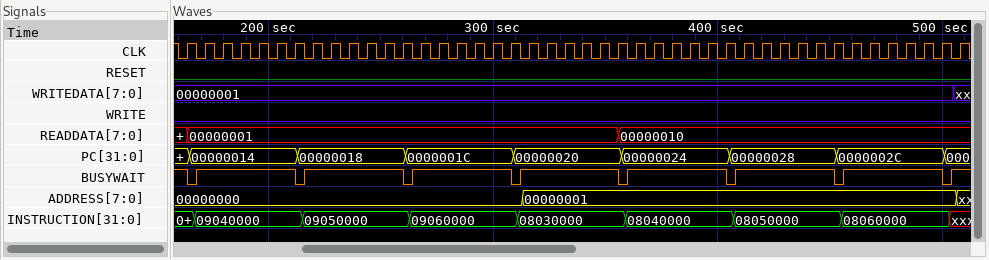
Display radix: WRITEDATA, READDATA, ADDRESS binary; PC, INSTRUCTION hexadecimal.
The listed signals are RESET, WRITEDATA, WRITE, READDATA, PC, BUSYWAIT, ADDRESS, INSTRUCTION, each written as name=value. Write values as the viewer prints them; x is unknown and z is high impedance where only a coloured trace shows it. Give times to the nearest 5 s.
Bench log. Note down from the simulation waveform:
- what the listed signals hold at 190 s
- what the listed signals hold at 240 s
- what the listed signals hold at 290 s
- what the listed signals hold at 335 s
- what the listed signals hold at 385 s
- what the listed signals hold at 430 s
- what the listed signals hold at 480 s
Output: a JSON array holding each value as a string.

["RESET=0, WRITEDATA=00000001, WRITE=0, READDATA=00000001, PC=00000014, BUSYWAIT=1, ADDRESS=00000000, INSTRUCTION=09040000", "RESET=0, WRITEDATA=00000001, WRITE=0, READDATA=00000001, PC=00000018, BUSYWAIT=1, ADDRESS=00000000, INSTRUCTION=09050000", "RESET=0, WRITEDATA=00000001, WRITE=0, READDATA=00000001, PC=0000001C, BUSYWAIT=1, ADDRESS=00000000, INSTRUCTION=09060000", "RESET=0, WRITEDATA=00000001, WRITE=0, READDATA=00000001, PC=00000020, BUSYWAIT=1, ADDRESS=00000001, INSTRUCTION=08030000", "RESET=0, WRITEDATA=00000001, WRITE=0, READDATA=00000010, PC=00000024, BUSYWAIT=1, ADDRESS=00000001, INSTRUCTION=08040000", "RESET=0, WRITEDATA=00000001, WRITE=0, READDATA=00000010, PC=00000028, BUSYWAIT=1, ADDRESS=00000001, INSTRUCTION=08050000", "RESET=0, WRITEDATA=00000001, WRITE=0, READDATA=00000010, PC=0000002C, BUSYWAIT=1, ADDRESS=00000001, INSTRUCTION=08060000"]
